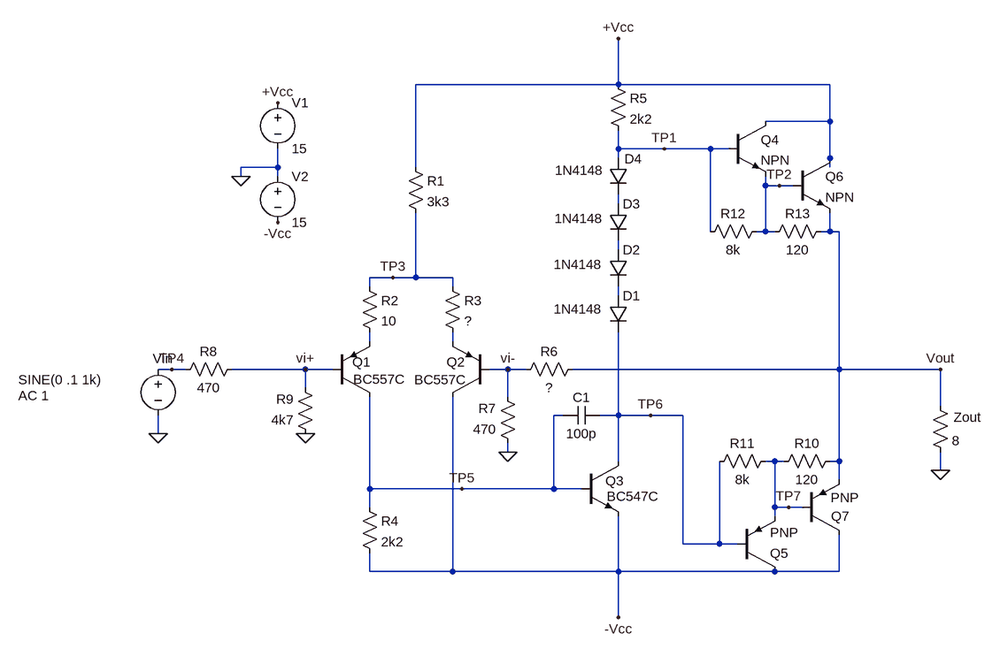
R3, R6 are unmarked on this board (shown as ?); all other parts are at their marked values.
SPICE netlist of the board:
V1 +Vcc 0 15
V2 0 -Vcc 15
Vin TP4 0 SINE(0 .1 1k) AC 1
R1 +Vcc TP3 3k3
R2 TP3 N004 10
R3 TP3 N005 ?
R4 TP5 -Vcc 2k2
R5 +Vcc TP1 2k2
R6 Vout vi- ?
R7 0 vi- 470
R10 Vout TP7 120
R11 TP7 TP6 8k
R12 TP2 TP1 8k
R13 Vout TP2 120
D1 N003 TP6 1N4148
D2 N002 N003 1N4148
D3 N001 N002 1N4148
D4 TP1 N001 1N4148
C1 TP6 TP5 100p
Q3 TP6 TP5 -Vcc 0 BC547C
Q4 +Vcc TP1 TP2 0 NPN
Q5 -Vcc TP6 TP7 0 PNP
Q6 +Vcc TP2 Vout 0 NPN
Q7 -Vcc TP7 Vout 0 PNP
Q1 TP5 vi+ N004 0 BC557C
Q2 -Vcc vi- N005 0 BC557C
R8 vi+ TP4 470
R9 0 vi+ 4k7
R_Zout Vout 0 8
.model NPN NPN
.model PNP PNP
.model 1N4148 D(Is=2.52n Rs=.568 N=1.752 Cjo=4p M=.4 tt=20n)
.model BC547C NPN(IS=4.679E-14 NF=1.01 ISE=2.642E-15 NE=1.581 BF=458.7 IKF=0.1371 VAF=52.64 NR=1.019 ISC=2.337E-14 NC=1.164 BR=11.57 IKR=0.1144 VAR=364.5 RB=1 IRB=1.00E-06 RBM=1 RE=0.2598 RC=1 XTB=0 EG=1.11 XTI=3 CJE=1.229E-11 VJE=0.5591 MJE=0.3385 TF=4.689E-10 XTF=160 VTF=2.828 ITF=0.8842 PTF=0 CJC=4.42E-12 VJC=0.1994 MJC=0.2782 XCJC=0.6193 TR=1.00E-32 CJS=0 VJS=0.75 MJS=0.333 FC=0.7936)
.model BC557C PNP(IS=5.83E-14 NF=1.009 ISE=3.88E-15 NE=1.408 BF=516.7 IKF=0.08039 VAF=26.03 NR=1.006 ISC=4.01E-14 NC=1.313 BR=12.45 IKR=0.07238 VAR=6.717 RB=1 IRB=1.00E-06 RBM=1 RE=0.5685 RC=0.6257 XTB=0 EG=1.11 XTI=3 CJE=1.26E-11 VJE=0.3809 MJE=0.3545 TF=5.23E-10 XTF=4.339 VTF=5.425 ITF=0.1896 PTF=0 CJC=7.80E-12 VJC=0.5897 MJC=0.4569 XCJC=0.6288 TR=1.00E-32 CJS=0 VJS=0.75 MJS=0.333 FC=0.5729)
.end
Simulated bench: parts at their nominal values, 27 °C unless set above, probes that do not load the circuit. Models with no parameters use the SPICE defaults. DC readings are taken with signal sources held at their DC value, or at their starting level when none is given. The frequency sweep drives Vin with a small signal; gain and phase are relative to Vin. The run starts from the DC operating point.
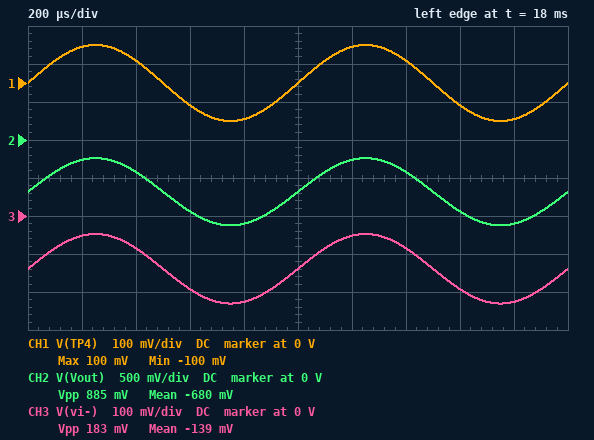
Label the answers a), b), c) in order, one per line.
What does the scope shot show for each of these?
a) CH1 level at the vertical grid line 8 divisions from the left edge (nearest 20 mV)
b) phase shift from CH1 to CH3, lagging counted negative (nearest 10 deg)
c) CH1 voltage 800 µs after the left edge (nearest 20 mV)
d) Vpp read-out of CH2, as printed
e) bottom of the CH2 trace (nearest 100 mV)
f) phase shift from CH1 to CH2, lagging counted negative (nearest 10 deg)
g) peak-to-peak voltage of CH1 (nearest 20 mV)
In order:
a) -60 mV
b) 0 deg
c) -100 mV
d) 885 mV
e) -1.1 V
f) 0 deg
g) 200 mV
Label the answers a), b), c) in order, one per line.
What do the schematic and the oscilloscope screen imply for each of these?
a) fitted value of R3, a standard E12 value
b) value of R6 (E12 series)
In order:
a) 18 Ω
b) 1.8 kΩ
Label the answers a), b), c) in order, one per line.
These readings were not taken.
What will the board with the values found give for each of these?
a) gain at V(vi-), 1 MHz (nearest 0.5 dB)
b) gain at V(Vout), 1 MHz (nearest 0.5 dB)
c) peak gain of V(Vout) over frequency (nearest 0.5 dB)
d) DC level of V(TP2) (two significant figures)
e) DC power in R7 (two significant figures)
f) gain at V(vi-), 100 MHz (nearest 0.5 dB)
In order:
a) -1.0 dB
b) 12.5 dB
c) 13.0 dB
d) -490 mV
e) 41 µW
f) -13.0 dB
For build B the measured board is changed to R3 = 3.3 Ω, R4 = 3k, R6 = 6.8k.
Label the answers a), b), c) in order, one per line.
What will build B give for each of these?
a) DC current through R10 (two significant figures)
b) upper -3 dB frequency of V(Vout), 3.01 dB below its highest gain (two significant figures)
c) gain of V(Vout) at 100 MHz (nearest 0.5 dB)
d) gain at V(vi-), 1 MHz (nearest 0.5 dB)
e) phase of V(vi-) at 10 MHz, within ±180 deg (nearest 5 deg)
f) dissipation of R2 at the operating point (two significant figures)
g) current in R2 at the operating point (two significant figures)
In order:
a) 7.6 mA
b) 800 kHz
c) -37.5 dB
d) -5.0 dB
e) 65 deg
f) 560 nW
g) 240 µA
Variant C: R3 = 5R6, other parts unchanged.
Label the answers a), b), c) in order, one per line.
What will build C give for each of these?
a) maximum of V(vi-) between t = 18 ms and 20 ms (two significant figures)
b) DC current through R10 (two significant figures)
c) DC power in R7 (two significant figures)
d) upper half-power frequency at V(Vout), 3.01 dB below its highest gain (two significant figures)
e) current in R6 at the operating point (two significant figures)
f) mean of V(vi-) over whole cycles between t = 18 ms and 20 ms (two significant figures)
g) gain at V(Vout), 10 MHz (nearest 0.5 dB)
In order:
a) 2.4 mV
b) 7.3 mA
c) 17 µW
d) 3.8 MHz
e) 190 µA
f) -89 mV
g) 0 dB
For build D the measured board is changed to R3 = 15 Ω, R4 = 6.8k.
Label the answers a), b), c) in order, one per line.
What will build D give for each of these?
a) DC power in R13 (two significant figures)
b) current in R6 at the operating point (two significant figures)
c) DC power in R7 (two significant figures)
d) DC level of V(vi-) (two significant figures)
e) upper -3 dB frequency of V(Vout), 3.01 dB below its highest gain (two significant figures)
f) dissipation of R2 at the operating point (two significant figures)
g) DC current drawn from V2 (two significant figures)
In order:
a) 300 µW
b) 350 µA
c) 55 µW
d) -160 mV
e) 1.3 MHz
f) 120 nW
g) 110 mA
